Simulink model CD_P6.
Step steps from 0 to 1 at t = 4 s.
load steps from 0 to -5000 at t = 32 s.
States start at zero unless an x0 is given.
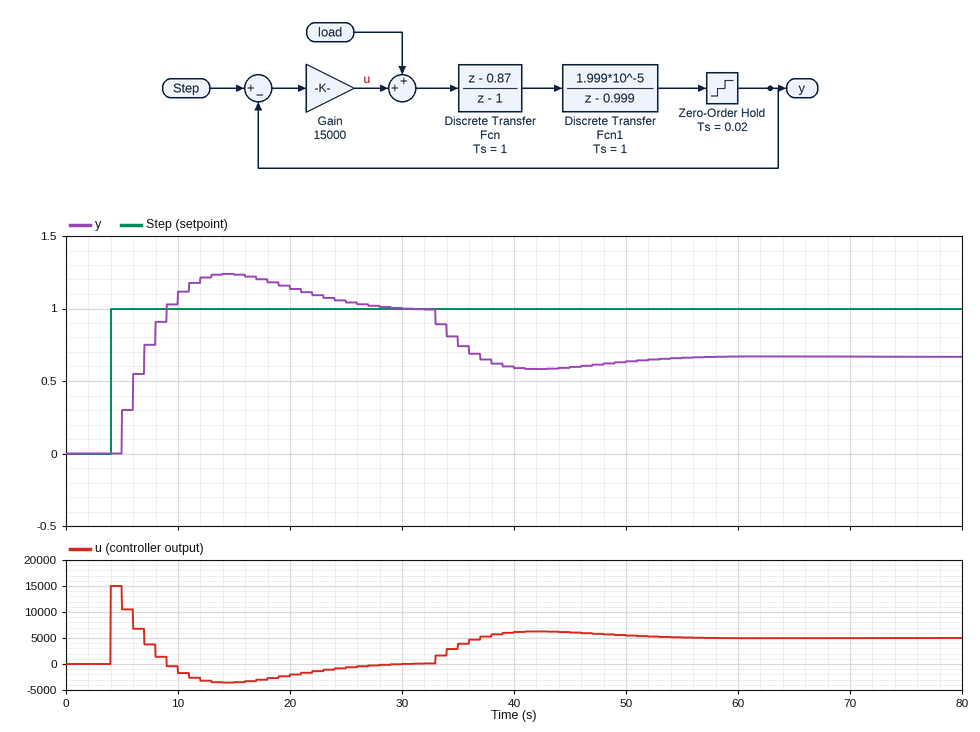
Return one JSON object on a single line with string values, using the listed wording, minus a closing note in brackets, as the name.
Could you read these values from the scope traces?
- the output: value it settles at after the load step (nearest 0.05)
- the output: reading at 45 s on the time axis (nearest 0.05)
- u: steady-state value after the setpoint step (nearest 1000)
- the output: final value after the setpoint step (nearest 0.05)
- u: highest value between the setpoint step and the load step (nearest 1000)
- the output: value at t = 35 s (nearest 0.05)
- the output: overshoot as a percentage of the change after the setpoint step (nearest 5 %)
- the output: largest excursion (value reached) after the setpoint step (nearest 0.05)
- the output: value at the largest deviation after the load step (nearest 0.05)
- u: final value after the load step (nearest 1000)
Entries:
{"the output: value it settles at after the load step": "0.65", "the output: reading at 45 s on the time axis": "0.60", "u: steady-state value after the setpoint step": "0", "the output: final value after the setpoint step": "1.00", "u: highest value between the setpoint step and the load step": "15000", "the output: value at t = 35 s": "0.75", "the output: overshoot as a percentage of the change after the setpoint step": "25 %", "the output: largest excursion (value reached) after the setpoint step": "1.25", "the output: value at the largest deviation after the load step": "0.60", "u: final value after the load step": "5000"}
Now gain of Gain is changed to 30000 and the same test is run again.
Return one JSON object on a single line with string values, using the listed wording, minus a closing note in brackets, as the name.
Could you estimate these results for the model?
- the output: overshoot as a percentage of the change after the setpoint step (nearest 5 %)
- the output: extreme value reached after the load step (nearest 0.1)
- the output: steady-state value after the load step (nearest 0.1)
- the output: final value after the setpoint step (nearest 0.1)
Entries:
{"the output: overshoot as a percentage of the change after the setpoint step": "15 %", "the output: extreme value reached after the load step": "0.8", "the output: steady-state value after the load step": "0.8", "the output: final value after the setpoint step": "1.0"}
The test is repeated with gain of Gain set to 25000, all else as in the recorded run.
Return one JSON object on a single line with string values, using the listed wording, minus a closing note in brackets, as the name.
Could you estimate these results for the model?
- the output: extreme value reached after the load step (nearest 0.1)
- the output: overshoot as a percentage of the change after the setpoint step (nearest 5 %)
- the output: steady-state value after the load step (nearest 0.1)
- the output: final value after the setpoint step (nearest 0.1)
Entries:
{"the output: extreme value reached after the load step": "0.8", "the output: overshoot as a percentage of the change after the setpoint step": "20 %", "the output: steady-state value after the load step": "0.8", "the output: final value after the setpoint step": "1.0"}
